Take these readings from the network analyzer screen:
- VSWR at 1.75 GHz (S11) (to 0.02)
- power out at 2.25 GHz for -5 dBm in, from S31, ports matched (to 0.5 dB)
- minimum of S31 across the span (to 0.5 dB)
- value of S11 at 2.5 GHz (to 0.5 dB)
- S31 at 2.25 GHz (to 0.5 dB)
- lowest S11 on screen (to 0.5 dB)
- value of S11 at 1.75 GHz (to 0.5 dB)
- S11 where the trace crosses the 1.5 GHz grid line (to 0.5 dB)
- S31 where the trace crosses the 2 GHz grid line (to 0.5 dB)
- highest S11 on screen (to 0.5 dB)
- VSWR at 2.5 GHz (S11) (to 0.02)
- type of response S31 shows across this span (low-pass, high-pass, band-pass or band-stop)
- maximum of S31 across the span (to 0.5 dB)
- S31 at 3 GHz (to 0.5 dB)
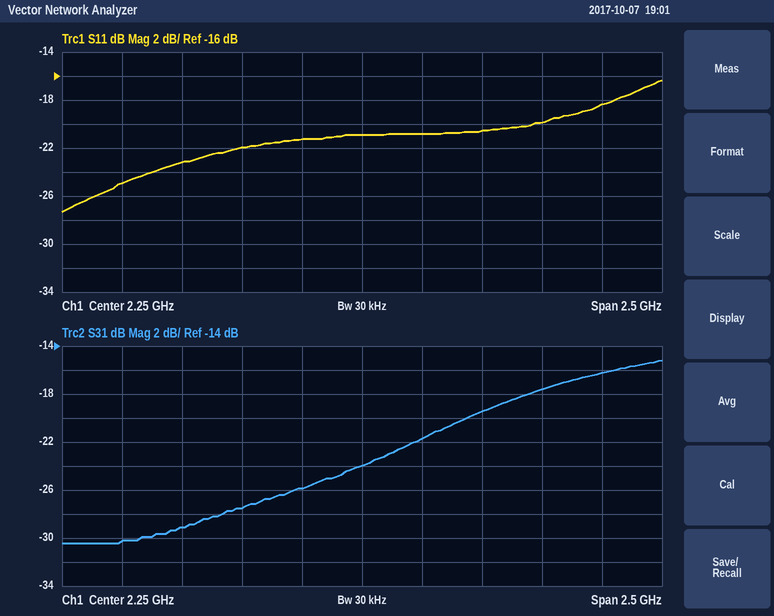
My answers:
1.18
-29.0 dBm
-30.5 dB
-21.0 dB
-24.0 dB
-27.5 dB
-22.0 dB
-23.0 dB
-26.0 dB
-16.5 dB
1.20
high-pass
-15.0 dB
-17.5 dB
